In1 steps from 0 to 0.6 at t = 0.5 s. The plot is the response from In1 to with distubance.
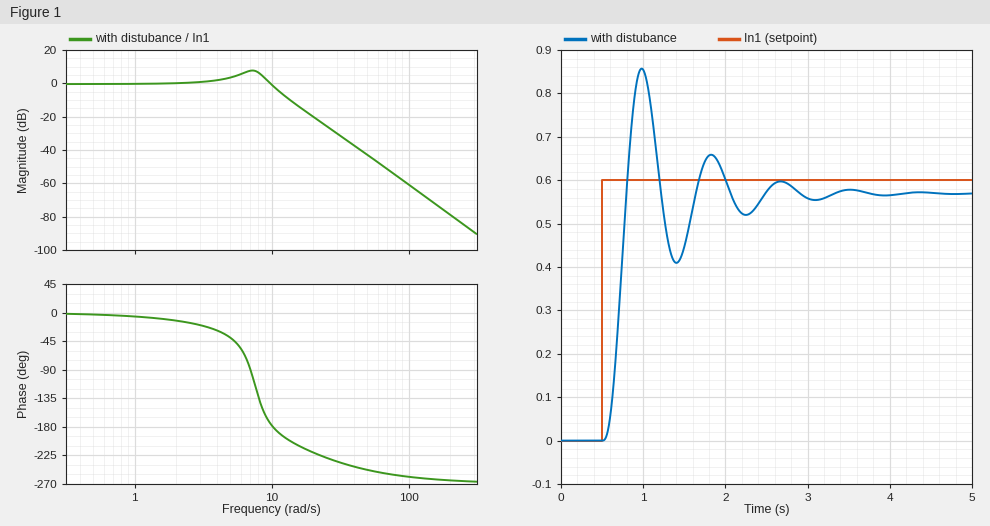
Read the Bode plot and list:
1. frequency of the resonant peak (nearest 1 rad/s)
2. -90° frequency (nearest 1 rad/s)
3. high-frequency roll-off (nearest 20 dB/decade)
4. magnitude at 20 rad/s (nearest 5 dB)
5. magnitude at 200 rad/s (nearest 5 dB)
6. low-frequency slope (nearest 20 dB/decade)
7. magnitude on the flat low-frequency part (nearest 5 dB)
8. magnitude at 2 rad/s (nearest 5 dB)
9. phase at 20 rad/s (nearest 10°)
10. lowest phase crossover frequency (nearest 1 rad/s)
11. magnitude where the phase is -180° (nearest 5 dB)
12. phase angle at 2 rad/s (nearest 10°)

7 rad/s
7 rad/s
-60 dB/decade
-20 dB
-80 dB
0 dB/decade
0 dB
0 dB
-220°
10 rad/s
0 dB
-10°
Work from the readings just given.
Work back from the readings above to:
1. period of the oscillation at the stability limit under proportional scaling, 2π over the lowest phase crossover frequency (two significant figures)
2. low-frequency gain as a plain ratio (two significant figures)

0.63 s
1.0
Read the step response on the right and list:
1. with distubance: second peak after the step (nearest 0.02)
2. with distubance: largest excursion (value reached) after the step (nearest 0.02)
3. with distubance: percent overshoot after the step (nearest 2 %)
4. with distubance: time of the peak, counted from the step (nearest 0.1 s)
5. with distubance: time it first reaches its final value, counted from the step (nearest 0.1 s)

0.66
0.86
50 %
0.5 s
0.3 s
